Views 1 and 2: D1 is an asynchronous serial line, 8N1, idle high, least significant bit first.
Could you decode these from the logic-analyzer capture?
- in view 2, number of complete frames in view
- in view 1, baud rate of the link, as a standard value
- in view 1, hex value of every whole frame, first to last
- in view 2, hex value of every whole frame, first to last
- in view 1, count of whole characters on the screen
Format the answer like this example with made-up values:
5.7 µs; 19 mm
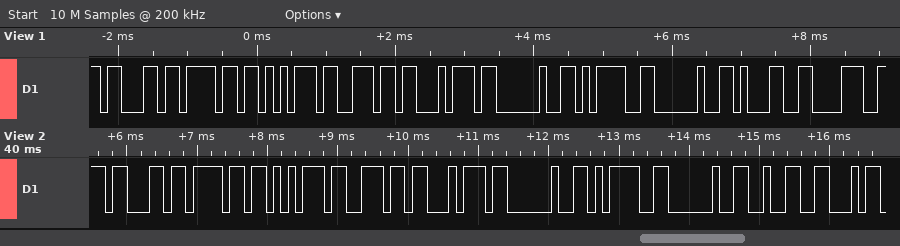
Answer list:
9; 9600 baud; 63 6F 75 6E 74 20 3D 20 31 38; 63 6F 75 6E 74 20 3D 20 32; 10
